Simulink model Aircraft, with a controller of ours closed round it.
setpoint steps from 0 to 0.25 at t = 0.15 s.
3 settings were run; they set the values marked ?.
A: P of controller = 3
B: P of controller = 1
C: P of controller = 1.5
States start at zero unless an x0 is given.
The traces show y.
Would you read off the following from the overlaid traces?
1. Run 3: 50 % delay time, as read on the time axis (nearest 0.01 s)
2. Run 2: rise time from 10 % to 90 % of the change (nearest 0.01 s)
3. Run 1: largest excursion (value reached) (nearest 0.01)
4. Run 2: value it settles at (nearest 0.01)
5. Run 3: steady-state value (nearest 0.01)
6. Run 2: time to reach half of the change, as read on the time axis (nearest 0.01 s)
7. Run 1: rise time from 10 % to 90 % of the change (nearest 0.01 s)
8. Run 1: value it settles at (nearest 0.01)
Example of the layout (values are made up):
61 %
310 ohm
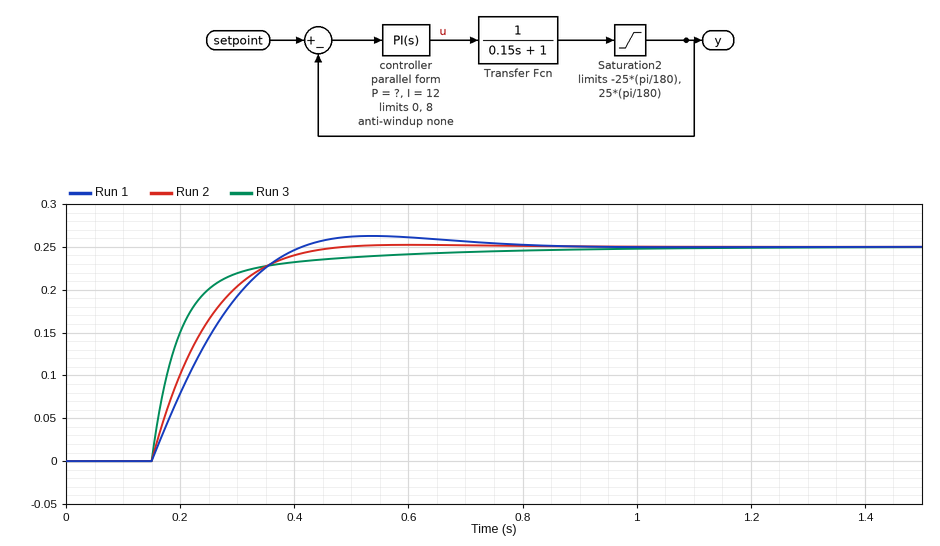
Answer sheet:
0.19 s
0.18 s
0.26
0.25
0.25
0.22 s
0.18 s
0.25
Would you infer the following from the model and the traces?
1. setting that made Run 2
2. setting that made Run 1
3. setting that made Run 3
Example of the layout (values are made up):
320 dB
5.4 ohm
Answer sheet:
C
B
A
